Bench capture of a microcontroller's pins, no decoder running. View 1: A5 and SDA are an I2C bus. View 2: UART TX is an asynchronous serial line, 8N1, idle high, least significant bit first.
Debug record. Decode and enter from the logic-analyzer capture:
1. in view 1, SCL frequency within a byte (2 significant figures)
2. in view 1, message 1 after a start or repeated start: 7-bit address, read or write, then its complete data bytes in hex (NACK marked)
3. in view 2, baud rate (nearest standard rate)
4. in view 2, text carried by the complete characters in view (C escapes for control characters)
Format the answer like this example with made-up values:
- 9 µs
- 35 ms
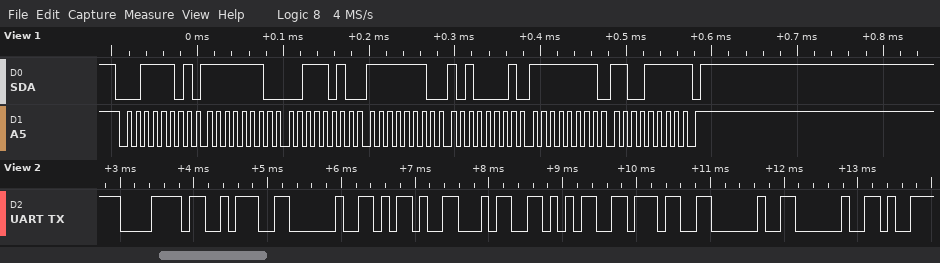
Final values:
- 100 kHz
- 0x1E read: FE 3A FE A1 FF CF NACK
- 9600 baud
- "x: -457  "
